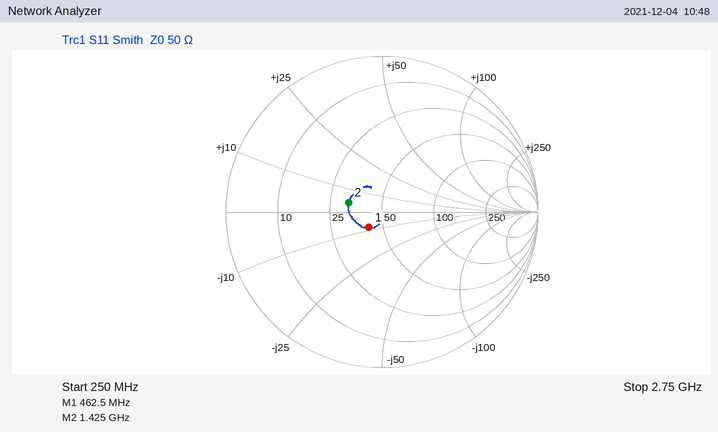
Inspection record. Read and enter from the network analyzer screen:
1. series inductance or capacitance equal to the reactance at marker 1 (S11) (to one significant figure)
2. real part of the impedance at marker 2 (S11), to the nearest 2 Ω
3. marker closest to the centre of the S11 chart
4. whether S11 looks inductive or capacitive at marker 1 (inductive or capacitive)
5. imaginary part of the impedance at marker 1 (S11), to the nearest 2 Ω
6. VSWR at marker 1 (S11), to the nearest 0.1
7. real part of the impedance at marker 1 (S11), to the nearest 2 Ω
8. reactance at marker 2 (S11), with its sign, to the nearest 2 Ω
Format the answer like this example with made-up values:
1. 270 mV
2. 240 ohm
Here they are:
1. 40 pF
2. 32 Ω
3. marker 1
4. capacitive
5. -8 Ω
6. 1.3
7. 42 Ω
8. +4 Ω
